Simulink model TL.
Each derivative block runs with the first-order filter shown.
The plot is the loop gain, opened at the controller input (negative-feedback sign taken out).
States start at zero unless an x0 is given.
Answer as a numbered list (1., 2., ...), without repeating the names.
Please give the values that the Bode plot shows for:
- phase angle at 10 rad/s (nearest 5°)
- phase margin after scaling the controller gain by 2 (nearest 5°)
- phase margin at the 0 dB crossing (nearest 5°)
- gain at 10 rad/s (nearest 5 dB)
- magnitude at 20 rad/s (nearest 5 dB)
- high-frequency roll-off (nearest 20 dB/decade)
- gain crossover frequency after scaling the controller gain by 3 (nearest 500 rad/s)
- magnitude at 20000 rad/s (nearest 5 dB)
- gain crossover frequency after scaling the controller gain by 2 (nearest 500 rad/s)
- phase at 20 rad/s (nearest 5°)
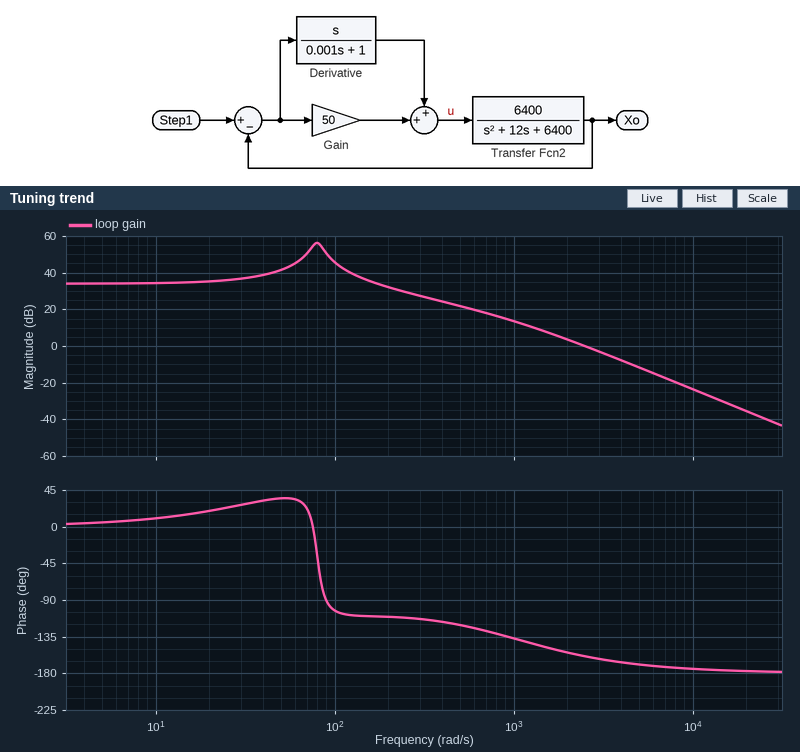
1. 10°
2. 15°
3. 20°
4. 35 dB
5. 35 dB
6. -40 dB/decade
7. 4500 rad/s
8. -35 dB
9. 3500 rad/s
10. 20°
